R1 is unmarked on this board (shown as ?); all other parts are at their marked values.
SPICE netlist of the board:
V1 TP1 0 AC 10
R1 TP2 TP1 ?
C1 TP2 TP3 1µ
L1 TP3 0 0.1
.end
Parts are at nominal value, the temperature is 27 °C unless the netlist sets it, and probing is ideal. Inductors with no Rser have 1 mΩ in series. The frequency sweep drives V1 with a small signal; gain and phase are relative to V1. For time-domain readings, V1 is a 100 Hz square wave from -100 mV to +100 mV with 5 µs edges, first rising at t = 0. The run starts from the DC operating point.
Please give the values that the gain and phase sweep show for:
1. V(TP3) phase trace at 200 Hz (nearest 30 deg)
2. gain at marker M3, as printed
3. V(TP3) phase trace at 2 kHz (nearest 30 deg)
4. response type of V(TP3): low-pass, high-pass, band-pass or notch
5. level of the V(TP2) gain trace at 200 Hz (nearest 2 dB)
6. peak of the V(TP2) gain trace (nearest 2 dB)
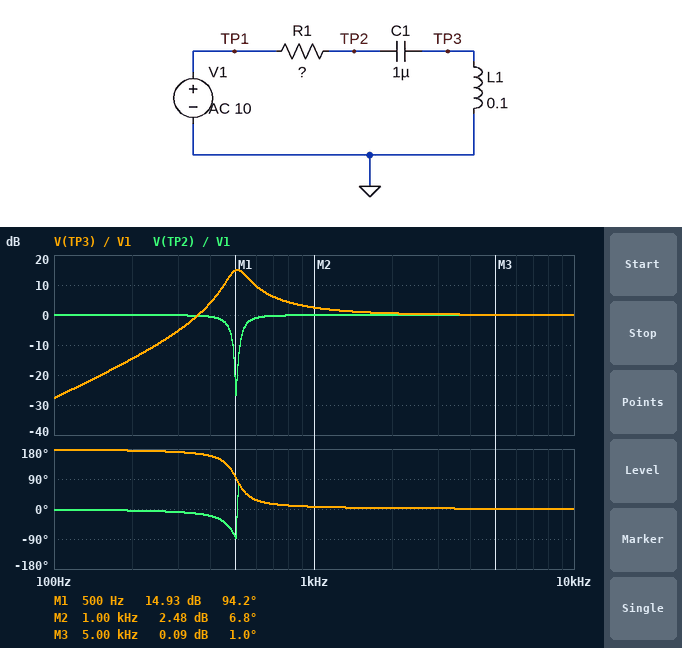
180 deg
0.09 dB
0 deg
high-pass
0 dB
0 dB
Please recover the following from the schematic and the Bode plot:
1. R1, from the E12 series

56 Ω
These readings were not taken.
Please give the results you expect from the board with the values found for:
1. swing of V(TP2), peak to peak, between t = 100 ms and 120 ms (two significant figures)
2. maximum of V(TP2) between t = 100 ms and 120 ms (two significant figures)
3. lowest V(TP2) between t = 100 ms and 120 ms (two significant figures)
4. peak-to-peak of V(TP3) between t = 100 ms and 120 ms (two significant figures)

260 mV
130 mV
-130 mV
530 mV
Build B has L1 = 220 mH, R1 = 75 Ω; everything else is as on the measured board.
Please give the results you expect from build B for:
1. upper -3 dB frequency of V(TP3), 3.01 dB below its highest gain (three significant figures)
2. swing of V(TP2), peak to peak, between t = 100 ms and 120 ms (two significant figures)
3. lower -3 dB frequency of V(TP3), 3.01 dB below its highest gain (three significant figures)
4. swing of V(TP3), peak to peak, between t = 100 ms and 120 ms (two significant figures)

373 Hz
250 mV
317 Hz
370 mV
